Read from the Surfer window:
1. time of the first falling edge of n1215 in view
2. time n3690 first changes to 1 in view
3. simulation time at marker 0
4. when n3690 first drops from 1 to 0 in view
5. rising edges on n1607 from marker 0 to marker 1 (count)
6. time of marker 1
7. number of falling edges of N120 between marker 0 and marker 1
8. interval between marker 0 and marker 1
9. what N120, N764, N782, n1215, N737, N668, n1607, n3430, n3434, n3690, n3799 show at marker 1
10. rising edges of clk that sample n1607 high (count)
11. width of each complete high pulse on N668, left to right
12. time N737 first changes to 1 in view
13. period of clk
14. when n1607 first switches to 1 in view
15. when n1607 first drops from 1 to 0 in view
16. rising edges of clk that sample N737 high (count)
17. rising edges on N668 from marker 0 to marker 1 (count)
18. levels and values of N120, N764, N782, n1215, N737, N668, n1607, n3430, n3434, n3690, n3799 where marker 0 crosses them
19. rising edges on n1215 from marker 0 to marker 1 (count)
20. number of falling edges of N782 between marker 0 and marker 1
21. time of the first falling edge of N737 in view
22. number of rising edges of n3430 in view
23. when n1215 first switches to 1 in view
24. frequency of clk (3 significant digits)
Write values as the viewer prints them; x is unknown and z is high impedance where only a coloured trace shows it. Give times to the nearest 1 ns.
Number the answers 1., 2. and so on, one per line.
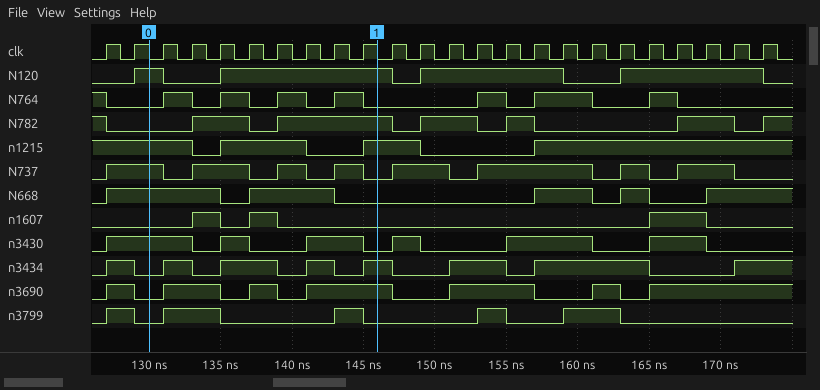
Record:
1. 133 ns
2. 127 ns
3. 130 ns
4. 129 ns
5. 2
6. 146 ns
7. 1
8. 16 ns
9. N120=1, N764=0, N782=1, n1215=1, N737=0, N668=0, n1607=0, n3430=0, n3434=1, n3690=1, n3799=0
10. 4
11. 8 ns, 6 ns, 4 ns, 2 ns
12. 127 ns
13. 2 ns
14. 133 ns
15. 135 ns
16. 15
17. 1
18. N120=1, N764=0, N782=0, n1215=1, N737=1, N668=1, n1607=0, n3430=1, n3434=0, n3690=0, n3799=0
19. 2
20. 1
21. 131 ns
22. 6
23. 135 ns
24. 500 MHz
